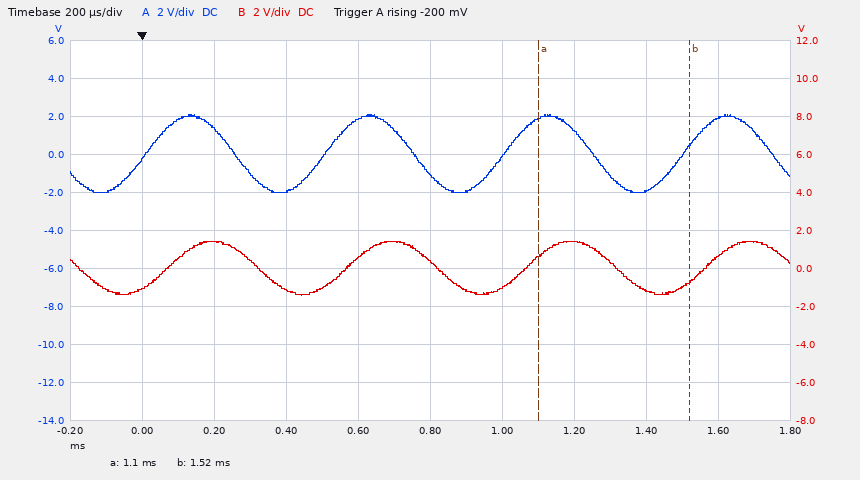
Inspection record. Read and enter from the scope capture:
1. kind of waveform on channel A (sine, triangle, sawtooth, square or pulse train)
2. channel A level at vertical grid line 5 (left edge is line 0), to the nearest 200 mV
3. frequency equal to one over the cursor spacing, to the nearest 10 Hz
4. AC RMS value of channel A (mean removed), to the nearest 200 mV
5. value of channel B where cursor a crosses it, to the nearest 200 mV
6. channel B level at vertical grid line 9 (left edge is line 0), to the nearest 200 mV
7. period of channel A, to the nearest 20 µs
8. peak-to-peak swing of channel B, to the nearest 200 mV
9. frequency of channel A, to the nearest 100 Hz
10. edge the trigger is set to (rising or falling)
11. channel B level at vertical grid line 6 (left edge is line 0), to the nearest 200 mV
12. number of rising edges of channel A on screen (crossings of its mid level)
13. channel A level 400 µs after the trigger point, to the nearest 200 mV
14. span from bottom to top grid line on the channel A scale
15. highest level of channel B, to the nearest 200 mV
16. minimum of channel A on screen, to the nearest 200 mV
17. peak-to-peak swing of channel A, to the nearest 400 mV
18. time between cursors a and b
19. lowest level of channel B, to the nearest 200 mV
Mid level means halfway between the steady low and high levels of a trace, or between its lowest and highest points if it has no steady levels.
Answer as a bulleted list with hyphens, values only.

- sine
- -1.0 V
- 2.38 kHz
- 1.4 V
- 600 mV
- 600 mV
- 500 µs
- 2.8 V
- 2.0 kHz
- rising
- -1.0 V
- 4
- -2.0 V
- 20 V
- 1.4 V
- -2.0 V
- 4.0 V
- 420 µs
- -1.4 V
